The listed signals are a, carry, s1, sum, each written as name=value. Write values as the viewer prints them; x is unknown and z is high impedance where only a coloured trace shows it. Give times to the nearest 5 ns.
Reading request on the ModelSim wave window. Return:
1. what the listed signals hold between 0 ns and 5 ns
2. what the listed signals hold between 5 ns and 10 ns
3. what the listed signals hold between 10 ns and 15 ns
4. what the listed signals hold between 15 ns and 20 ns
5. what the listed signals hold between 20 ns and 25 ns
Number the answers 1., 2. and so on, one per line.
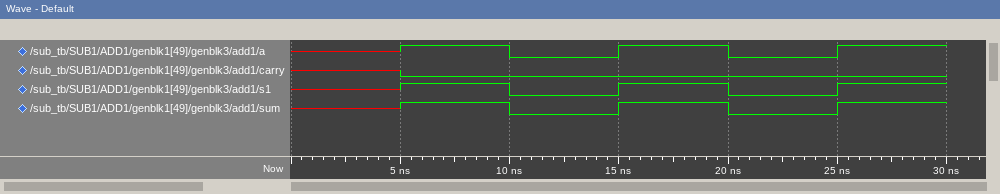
1. a=x, carry=x, s1=x, sum=x
2. a=1, carry=0, s1=1, sum=1
3. a=0, carry=0, s1=0, sum=0
4. a=1, carry=0, s1=1, sum=1
5. a=0, carry=0, s1=0, sum=0
